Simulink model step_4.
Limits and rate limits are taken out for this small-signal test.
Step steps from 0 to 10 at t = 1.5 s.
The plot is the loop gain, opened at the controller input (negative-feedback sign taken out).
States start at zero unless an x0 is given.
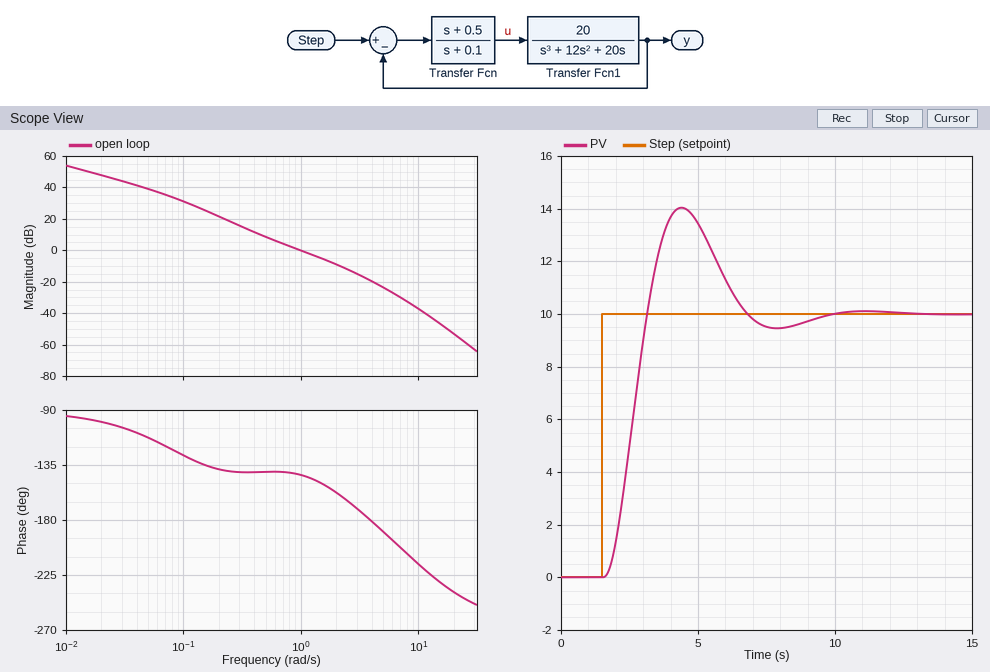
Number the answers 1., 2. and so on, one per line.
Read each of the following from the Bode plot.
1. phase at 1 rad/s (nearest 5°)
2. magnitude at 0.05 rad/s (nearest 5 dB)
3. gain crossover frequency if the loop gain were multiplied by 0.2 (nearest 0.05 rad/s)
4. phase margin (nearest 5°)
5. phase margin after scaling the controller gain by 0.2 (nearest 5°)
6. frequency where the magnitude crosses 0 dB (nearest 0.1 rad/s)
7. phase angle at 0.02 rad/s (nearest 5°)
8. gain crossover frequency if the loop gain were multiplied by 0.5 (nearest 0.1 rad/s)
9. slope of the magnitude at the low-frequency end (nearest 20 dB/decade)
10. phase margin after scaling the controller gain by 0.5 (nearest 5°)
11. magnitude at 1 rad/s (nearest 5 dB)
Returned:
1. -145°
2. 40 dB
3. 0.35 rad/s
4. 35°
5. 40°
6. 1.0 rad/s
7. -100°
8. 0.6 rad/s
9. -20 dB/decade
10. 40°
11. 0 dB
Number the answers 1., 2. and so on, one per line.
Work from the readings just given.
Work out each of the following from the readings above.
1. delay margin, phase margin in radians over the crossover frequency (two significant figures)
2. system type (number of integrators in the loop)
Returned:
1. 0.61 s
2. 1
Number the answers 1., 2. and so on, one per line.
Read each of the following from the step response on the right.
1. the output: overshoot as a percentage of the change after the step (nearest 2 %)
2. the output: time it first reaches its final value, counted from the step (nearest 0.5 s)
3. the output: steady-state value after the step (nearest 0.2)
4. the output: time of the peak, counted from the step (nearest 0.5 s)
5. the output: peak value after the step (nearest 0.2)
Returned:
1. 40 %
2. 1.5 s
3. 10.0
4. 3.0 s
5. 14.0
